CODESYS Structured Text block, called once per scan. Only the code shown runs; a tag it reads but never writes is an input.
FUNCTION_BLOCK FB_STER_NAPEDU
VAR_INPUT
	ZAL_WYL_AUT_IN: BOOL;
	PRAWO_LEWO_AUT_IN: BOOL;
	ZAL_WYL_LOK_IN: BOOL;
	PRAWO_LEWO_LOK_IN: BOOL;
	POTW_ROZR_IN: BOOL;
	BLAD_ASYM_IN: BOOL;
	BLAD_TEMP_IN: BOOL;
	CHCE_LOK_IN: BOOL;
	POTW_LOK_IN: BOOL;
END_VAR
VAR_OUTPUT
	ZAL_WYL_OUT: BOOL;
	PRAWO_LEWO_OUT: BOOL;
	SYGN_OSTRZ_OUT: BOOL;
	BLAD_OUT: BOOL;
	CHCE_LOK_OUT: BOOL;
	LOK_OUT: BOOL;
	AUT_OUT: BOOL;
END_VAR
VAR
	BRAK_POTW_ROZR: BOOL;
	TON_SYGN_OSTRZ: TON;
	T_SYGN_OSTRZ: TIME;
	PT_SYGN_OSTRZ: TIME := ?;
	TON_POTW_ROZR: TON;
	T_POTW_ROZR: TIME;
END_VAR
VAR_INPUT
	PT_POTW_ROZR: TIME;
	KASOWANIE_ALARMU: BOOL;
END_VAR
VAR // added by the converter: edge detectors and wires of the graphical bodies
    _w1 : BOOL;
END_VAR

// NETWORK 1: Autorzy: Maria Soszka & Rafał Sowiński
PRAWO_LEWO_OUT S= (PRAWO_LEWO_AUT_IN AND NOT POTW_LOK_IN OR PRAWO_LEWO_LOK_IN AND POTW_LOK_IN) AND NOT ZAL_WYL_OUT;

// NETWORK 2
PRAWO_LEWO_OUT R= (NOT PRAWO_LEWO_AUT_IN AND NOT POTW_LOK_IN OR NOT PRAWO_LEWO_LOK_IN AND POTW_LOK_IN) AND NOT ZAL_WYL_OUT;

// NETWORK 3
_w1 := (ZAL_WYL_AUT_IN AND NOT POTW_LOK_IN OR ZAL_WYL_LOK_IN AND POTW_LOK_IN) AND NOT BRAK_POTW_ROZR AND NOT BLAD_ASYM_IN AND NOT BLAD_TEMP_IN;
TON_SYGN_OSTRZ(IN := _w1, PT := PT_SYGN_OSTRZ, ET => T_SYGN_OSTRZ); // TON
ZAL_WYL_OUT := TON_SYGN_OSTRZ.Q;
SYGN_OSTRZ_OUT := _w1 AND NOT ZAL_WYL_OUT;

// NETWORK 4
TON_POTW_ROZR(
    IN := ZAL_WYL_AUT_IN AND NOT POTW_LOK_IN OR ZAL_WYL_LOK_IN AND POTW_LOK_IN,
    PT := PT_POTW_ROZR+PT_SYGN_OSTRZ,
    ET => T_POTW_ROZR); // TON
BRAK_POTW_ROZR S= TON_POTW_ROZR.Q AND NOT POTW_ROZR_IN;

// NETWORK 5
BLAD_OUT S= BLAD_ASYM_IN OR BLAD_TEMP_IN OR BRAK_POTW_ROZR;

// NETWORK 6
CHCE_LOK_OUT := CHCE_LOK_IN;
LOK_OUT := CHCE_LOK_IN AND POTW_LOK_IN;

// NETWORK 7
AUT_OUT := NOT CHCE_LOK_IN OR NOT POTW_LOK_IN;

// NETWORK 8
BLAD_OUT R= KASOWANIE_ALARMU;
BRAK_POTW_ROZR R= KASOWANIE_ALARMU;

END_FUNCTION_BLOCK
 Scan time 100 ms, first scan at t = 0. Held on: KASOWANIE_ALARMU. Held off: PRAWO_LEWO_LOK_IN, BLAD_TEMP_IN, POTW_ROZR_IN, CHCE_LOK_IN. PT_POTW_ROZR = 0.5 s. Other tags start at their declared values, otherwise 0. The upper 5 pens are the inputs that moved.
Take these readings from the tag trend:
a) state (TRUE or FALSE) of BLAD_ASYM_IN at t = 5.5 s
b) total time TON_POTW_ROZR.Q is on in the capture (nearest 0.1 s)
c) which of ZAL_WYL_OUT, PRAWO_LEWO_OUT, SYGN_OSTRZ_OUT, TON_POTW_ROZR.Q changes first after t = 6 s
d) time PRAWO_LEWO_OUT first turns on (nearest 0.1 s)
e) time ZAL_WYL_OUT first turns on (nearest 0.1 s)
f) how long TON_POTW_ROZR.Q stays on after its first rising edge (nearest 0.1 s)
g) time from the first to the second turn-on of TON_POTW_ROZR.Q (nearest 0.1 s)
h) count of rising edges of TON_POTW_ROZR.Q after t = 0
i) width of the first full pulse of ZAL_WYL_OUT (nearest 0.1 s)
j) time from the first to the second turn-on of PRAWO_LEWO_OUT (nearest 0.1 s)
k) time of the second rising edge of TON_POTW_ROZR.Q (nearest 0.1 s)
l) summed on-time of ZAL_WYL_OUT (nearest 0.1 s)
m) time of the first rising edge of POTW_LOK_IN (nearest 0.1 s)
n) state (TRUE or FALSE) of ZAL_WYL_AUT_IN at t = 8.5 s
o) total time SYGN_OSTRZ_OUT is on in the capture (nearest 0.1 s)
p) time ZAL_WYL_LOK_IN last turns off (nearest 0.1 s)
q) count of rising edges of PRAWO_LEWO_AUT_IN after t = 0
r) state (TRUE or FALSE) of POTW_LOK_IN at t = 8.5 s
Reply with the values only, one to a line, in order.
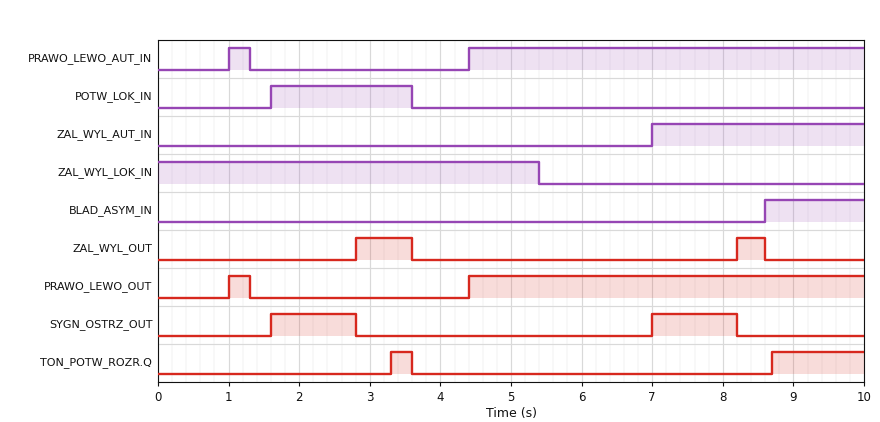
FALSE
1.6 s
SYGN_OSTRZ_OUT
1.0 s
2.8 s
0.3 s
5.4 s
2
0.8 s
3.4 s
8.7 s
1.2 s
1.6 s
TRUE
2.4 s
5.4 s
2
FALSE
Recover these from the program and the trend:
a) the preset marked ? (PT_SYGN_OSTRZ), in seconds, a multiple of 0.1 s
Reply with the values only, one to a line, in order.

1.2 s
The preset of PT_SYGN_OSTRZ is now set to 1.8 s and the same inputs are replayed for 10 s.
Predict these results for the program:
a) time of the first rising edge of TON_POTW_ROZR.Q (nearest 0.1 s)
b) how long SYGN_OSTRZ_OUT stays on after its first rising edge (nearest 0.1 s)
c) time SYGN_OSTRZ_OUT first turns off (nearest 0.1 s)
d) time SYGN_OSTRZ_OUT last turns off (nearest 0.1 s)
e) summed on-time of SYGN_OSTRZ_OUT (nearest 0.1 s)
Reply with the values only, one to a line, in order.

9.3 s
1.8 s
3.4 s
8.6 s
3.4 s
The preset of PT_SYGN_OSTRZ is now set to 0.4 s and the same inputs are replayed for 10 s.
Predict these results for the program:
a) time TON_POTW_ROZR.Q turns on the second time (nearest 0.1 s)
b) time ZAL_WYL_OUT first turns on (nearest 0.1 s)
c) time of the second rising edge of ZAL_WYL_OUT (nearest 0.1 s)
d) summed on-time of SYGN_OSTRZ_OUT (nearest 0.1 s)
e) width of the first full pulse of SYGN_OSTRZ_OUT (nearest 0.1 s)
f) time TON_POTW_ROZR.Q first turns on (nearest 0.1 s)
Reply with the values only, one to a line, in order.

7.9 s
2.0 s
7.4 s
0.8 s
0.4 s
2.5 s
